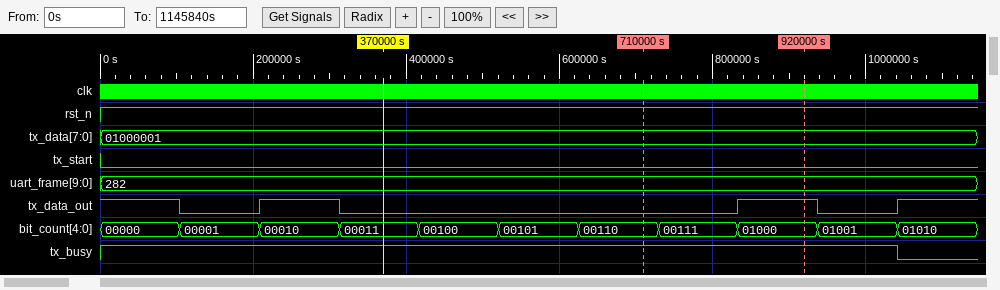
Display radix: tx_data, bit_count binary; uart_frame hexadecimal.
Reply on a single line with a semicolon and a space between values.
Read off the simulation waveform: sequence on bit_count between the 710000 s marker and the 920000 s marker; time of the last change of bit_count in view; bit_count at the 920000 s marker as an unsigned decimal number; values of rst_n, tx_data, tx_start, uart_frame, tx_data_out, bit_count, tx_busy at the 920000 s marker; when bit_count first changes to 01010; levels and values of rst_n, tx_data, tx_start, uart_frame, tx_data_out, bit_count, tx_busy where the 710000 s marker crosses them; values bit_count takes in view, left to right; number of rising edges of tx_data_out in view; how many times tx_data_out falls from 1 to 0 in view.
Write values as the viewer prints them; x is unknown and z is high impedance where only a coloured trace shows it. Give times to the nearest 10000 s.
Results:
00110, 00111, 01000; 1040000 s; 8; rst_n=1, tx_data=01000001, tx_start=0, uart_frame=282, tx_data_out=1, bit_count=01000, tx_busy=1; 1040000 s; rst_n=1, tx_data=01000001, tx_start=0, uart_frame=282, tx_data_out=0, bit_count=00110, tx_busy=1; 00000, 00001, 00010, 00011, 00100, 00101, 00110, 00111, 01000, 01001, 01010; 3; 3
